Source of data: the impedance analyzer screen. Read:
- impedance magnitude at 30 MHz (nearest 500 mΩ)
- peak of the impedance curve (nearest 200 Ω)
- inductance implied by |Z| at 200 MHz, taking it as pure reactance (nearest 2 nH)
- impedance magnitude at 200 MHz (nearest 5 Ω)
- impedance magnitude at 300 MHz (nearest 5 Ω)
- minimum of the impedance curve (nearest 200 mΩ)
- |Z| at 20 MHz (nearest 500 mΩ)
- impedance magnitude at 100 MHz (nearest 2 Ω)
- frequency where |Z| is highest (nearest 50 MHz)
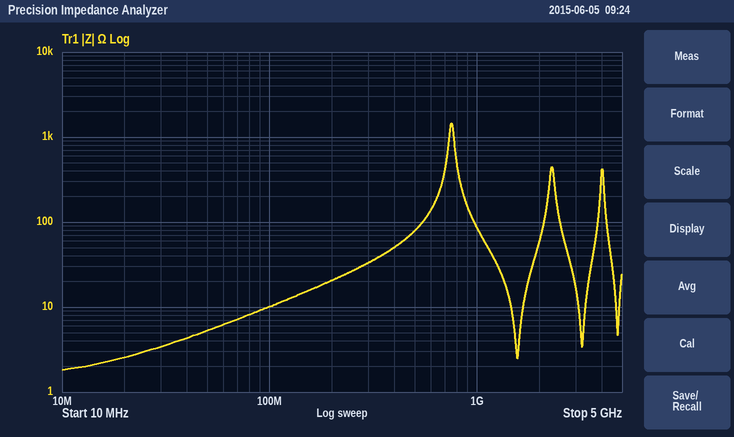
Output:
3.5 Ω
1.4 kΩ
16 nH
20 Ω
35 Ω
1.8 Ω
2.5 Ω
10 Ω
750 MHz
